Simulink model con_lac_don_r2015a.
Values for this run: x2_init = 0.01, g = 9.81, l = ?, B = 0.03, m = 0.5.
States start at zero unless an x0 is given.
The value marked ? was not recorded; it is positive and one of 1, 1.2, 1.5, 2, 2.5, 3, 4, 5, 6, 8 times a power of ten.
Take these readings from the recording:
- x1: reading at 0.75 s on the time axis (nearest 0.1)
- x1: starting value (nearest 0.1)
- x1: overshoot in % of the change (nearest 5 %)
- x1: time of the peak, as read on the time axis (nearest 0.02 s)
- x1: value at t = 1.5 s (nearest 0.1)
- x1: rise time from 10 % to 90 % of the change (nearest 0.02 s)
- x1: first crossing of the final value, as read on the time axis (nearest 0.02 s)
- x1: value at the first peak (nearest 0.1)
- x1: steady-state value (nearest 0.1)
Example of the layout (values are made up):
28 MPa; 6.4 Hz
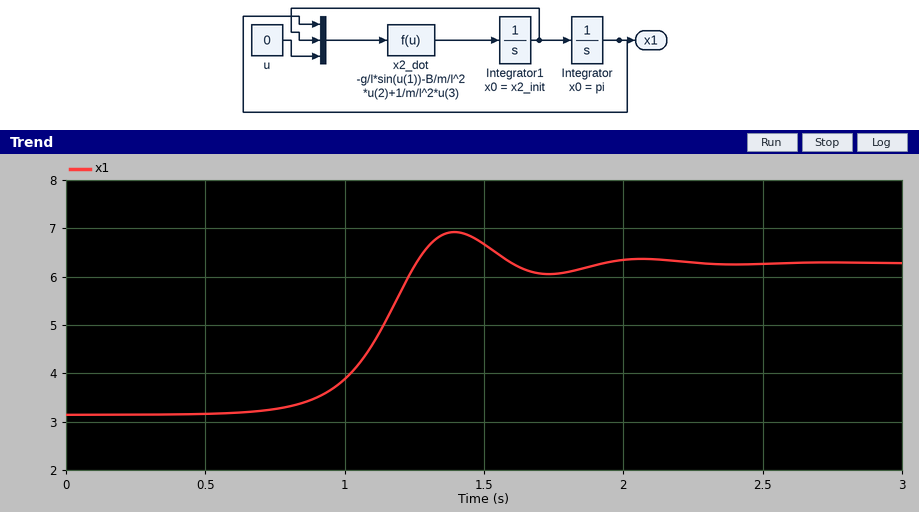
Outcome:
3.3; 3.1; 20 %; 1.40 s; 6.7; 0.34 s; 1.26 s; 6.9; 6.3
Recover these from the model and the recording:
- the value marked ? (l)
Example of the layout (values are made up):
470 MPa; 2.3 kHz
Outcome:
0.1
